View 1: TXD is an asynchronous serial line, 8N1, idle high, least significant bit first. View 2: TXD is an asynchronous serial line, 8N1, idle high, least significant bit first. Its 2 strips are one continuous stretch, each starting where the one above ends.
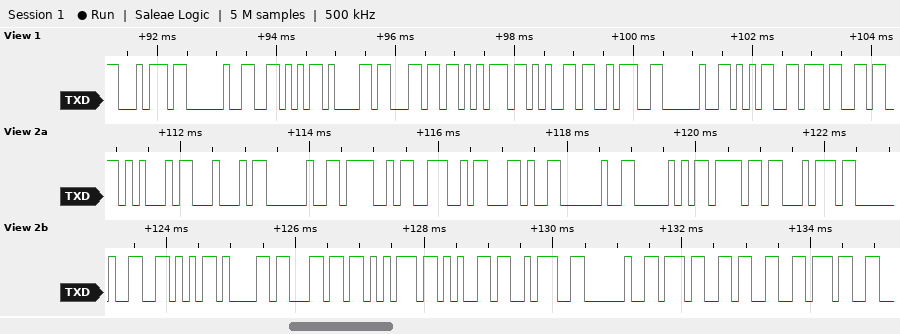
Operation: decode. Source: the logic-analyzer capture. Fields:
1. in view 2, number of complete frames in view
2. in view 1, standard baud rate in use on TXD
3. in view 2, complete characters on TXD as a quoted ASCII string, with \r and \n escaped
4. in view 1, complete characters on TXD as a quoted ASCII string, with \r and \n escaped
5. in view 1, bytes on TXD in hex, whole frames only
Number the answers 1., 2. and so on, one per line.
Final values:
1. 21
2. 9600 baud
3. "ED ON, Pot Value: 737"
4. "t Value: 57"
5. 74 20 56 61 6C 75 65 3A 20 35 37
